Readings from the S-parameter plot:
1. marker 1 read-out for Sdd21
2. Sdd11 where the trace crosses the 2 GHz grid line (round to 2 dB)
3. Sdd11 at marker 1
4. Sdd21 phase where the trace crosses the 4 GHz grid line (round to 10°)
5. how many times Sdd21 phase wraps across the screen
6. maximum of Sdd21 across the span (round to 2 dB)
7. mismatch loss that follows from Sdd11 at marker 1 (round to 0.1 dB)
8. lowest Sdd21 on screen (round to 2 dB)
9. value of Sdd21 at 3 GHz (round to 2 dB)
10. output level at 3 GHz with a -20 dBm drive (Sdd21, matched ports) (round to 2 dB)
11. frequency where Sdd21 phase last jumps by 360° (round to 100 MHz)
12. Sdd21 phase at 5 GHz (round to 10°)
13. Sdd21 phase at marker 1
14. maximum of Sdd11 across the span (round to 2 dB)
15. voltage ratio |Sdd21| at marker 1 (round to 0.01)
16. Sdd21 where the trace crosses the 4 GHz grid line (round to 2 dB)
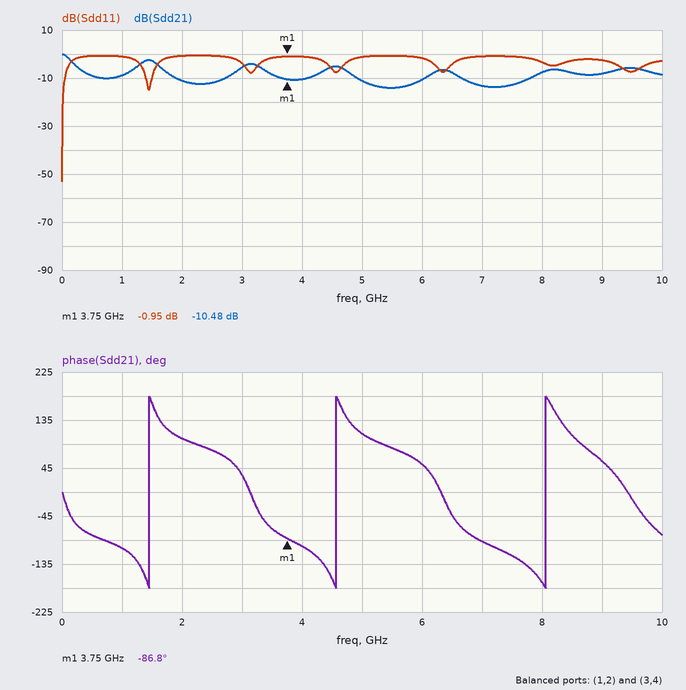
-10.48 dB
0 dB
-0.95 dB
-100°
3
0 dB
7.1 dB
-14 dB
-6 dB
-26 dBm
8.1 GHz
110°
-86.8°
0 dB
0.30
-10 dB
